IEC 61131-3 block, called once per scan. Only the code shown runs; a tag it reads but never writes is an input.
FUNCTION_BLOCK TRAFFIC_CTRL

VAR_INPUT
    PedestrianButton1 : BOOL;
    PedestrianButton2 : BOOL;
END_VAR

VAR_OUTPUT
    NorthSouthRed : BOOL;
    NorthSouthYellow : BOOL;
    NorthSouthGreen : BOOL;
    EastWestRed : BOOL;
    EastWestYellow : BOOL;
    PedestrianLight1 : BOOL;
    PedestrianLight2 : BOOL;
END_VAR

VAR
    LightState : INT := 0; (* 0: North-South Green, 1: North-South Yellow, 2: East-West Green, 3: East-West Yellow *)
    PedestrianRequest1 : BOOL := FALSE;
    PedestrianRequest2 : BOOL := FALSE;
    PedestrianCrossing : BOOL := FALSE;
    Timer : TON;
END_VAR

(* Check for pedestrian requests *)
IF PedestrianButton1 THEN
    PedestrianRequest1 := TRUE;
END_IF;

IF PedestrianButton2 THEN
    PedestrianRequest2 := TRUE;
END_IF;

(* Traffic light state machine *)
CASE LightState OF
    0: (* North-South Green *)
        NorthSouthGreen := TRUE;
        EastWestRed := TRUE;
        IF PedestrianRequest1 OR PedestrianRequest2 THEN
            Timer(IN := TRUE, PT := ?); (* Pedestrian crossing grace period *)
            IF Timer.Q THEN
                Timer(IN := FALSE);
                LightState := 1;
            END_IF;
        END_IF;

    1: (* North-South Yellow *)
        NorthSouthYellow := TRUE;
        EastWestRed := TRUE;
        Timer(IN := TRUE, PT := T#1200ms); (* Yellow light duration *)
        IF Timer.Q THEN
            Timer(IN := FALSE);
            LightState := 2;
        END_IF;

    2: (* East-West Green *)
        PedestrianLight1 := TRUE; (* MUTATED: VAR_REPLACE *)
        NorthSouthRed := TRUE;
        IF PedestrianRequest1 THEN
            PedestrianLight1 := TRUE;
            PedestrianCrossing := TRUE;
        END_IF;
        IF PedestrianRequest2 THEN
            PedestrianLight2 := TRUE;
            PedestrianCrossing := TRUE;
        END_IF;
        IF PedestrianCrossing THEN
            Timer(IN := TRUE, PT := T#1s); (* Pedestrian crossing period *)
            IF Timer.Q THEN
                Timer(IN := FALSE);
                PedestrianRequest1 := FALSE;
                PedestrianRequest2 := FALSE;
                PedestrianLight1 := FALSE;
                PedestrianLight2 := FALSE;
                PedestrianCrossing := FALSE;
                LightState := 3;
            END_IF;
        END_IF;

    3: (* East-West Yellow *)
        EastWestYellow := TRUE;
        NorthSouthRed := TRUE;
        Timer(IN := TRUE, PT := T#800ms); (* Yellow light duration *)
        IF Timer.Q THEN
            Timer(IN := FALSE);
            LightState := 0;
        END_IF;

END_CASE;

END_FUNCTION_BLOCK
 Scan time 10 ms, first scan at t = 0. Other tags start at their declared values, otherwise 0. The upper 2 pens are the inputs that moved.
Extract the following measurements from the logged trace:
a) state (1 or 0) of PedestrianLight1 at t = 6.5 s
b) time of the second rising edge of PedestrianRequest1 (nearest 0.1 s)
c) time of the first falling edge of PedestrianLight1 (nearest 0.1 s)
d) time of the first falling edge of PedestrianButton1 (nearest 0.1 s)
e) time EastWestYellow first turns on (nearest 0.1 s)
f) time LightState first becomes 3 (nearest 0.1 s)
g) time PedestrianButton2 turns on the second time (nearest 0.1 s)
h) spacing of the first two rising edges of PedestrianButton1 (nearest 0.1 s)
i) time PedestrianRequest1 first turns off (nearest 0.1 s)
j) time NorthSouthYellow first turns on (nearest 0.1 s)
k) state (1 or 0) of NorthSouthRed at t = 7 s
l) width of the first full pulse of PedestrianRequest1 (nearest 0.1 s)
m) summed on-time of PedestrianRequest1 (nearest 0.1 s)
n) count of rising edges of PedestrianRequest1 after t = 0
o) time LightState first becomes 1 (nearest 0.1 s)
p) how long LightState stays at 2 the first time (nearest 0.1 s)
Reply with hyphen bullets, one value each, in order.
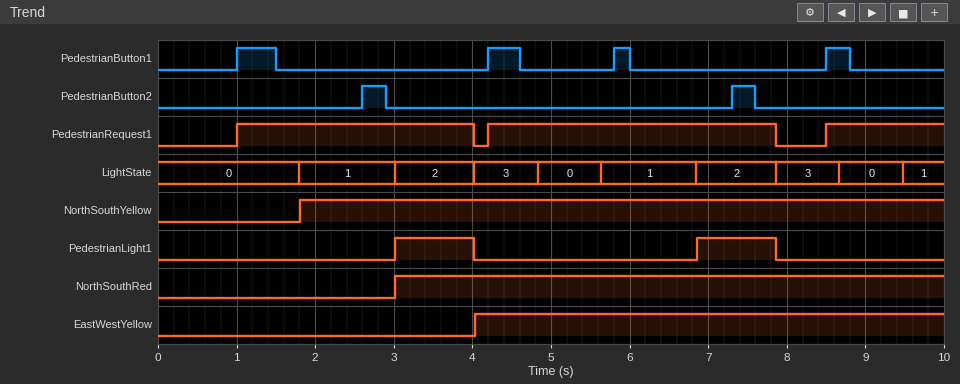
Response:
- 0
- 4.2 s
- 4.0 s
- 1.5 s
- 4.0 s
- 4.0 s
- 7.3 s
- 3.2 s
- 4.0 s
- 1.8 s
- 1
- 3.0 s
- 8.2 s
- 3
- 1.8 s
- 1.0 s
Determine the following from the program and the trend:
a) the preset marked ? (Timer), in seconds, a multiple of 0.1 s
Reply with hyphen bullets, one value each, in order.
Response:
- 0.8 s
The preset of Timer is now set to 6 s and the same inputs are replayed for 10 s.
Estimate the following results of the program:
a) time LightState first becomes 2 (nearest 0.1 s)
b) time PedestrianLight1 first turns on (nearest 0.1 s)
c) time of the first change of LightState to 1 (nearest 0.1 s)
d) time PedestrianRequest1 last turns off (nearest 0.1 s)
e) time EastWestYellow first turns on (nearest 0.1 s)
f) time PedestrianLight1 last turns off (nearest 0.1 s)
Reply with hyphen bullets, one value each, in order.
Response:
- 8.2 s
- 8.2 s
- 7.0 s
- 9.2 s
- 9.2 s
- 9.2 s
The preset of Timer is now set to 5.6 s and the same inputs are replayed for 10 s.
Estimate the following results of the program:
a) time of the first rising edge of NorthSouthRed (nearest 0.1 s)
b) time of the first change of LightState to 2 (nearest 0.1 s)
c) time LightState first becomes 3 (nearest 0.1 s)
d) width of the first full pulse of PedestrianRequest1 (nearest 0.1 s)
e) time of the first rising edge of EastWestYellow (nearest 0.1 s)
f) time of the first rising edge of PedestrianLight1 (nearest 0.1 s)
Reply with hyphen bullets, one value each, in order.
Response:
- 7.8 s
- 7.8 s
- 8.8 s
- 7.8 s
- 8.8 s
- 7.8 s
